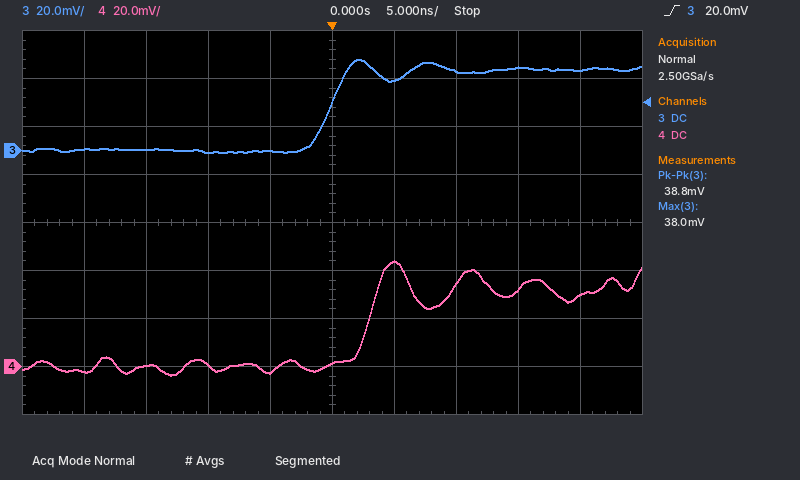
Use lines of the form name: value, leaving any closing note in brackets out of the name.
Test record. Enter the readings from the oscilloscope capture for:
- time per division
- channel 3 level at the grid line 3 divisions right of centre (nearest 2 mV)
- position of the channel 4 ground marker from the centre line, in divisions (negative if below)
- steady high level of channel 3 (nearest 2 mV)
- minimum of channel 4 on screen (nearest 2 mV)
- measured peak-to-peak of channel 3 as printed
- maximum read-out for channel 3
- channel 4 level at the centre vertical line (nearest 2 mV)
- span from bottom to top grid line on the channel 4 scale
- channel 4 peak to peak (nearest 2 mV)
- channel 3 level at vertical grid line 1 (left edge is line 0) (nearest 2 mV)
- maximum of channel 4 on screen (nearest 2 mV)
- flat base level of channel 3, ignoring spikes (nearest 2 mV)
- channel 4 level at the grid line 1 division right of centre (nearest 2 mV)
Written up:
time per division: 5 ns
channel 3 level at the grid line 3 divisions right of centre: 34 mV
position of the channel 4 ground marker from the centre line, in divisions: -3.0 div
steady high level of channel 3: 34 mV
minimum of channel 4 on screen: -4 mV
measured peak-to-peak of channel 3 as printed: 38.8 mV
maximum read-out for channel 3: 38.0 mV
channel 4 level at the centre vertical line: 2 mV
span from bottom to top grid line on the channel 4 scale: 160 mV
channel 4 peak to peak: 48 mV
channel 3 level at vertical grid line 1 (left edge is line 0): 0 mV
maximum of channel 4 on screen: 44 mV
flat base level of channel 3, ignoring spikes: 0 mV
channel 4 level at the grid line 1 division right of centre: 44 mV
